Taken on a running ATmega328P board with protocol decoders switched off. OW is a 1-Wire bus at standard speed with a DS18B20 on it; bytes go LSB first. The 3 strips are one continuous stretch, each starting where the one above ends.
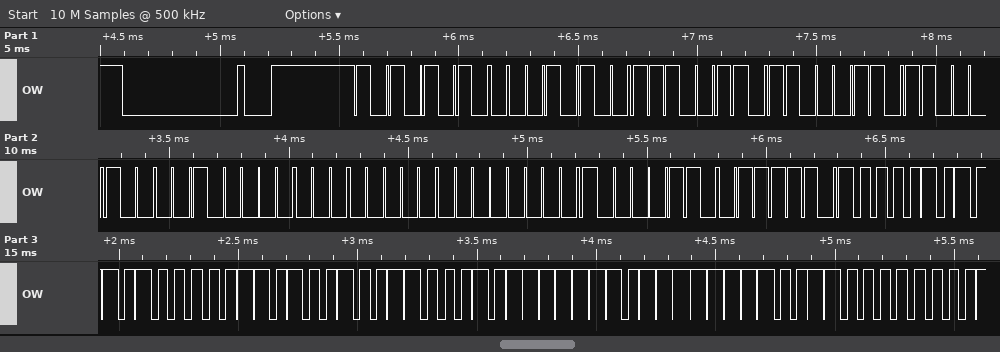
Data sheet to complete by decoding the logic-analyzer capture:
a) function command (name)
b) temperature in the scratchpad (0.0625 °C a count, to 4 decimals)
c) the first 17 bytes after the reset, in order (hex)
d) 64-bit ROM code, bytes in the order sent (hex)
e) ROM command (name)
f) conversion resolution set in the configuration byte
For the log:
Read Scratchpad
85.0000 °C
55 28 67 63 23 04 00 00 61 BE 50 05 4B 46 7F FF 0C
28 67 63 23 04 00 00 61
Match ROM
12 bits
